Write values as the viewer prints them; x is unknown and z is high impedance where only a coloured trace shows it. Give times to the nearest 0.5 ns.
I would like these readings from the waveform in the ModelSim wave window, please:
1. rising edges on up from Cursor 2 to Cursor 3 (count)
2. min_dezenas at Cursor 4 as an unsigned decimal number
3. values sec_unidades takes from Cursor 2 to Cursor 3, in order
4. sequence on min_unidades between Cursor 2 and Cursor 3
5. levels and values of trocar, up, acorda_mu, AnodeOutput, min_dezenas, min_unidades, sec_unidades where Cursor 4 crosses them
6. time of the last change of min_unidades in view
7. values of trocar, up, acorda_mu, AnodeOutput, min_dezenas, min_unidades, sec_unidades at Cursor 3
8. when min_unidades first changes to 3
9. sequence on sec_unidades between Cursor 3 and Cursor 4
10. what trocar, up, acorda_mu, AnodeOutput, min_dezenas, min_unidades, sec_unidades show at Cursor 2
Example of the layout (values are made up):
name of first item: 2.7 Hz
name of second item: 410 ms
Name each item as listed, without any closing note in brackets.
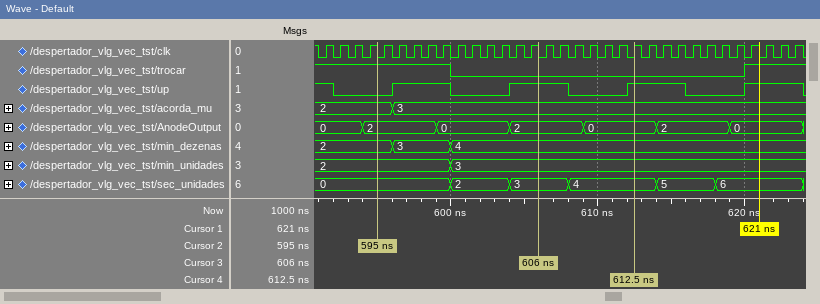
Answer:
rising edges on up from Cursor 2 to Cursor 3: 2
min_dezenas at Cursor 4 as an unsigned decimal number: 4
values sec_unidades takes from Cursor 2 to Cursor 3, in order: 0, 2, 3
sequence on min_unidades between Cursor 2 and Cursor 3: 2, 3
levels and values of trocar, up, acorda_mu, AnodeOutput, min_dezenas, min_unidades, sec_unidades where Cursor 4 crosses them: trocar=0, up=1, acorda_mu=3, AnodeOutput=0, min_dezenas=4, min_unidades=3, sec_unidades=4
time of the last change of min_unidades in view: 600 ns
values of trocar, up, acorda_mu, AnodeOutput, min_dezenas, min_unidades, sec_unidades at Cursor 3: trocar=0, up=1, acorda_mu=3, AnodeOutput=2, min_dezenas=4, min_unidades=3, sec_unidades=3
when min_unidades first changes to 3: 600 ns
sequence on sec_unidades between Cursor 3 and Cursor 4: 3, 4
what trocar, up, acorda_mu, AnodeOutput, min_dezenas, min_unidades, sec_unidades show at Cursor 2: trocar=1, up=0, acorda_mu=2, AnodeOutput=2, min_dezenas=2, min_unidades=2, sec_unidades=0
